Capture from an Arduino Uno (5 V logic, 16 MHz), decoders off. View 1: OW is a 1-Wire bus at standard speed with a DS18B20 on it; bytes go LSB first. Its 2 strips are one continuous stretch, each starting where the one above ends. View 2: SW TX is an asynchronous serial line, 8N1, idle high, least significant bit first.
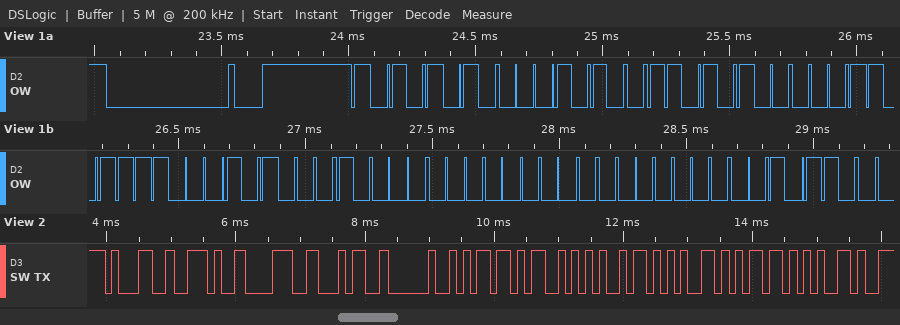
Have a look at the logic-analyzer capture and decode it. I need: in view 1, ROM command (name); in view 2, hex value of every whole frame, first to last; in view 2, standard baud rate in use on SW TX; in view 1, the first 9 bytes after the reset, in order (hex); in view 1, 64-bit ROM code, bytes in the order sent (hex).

Match ROM
0x31 0x2E 0x38 0x34 0x20 0x6D 0x53 0x69 0x65 0x6D 0x65
9600 baud
55 28 2B D8 A3 08 00 00 34
28 2B D8 A3 08 00 00 34
